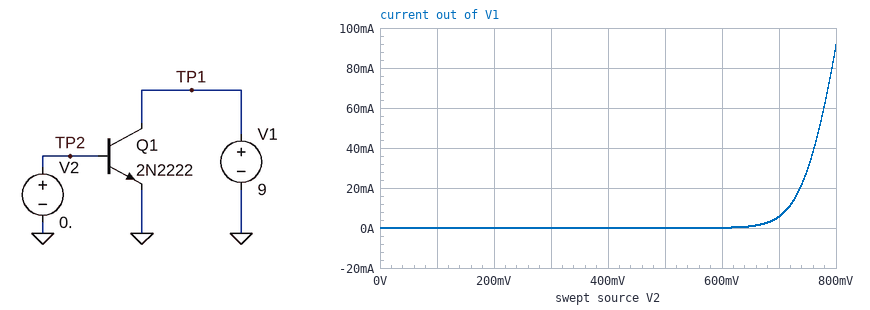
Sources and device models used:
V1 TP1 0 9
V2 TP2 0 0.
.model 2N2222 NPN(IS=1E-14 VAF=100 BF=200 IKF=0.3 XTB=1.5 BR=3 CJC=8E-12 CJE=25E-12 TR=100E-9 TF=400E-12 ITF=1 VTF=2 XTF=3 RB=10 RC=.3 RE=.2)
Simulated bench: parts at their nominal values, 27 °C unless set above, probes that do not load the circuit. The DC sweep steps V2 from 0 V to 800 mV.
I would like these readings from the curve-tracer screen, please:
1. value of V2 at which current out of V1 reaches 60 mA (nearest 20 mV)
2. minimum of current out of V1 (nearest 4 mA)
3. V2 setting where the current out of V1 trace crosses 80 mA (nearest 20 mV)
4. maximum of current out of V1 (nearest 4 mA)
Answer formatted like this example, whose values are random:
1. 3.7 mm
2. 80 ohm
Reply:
1. 780 mV
2. 0 A
3. 800 mV
4. 92 mA
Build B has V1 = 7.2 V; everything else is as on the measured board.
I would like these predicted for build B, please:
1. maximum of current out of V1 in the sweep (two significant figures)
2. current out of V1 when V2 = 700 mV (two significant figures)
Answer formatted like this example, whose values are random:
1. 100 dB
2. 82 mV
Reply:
1. 90 mA
2. 5.6 mA
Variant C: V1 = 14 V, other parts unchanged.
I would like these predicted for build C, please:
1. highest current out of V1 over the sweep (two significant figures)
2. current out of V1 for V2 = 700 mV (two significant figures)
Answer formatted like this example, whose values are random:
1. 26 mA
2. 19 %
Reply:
1. 94 mA
2. 6.0 mA
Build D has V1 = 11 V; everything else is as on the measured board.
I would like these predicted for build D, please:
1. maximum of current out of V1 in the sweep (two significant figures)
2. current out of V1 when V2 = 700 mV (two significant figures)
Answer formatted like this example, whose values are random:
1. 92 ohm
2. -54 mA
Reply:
1. 92 mA
2. 5.8 mA
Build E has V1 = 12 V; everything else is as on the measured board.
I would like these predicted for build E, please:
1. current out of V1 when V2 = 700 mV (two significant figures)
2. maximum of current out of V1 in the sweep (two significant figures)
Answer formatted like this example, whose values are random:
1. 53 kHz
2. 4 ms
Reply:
1. 5.9 mA
2. 93 mA
